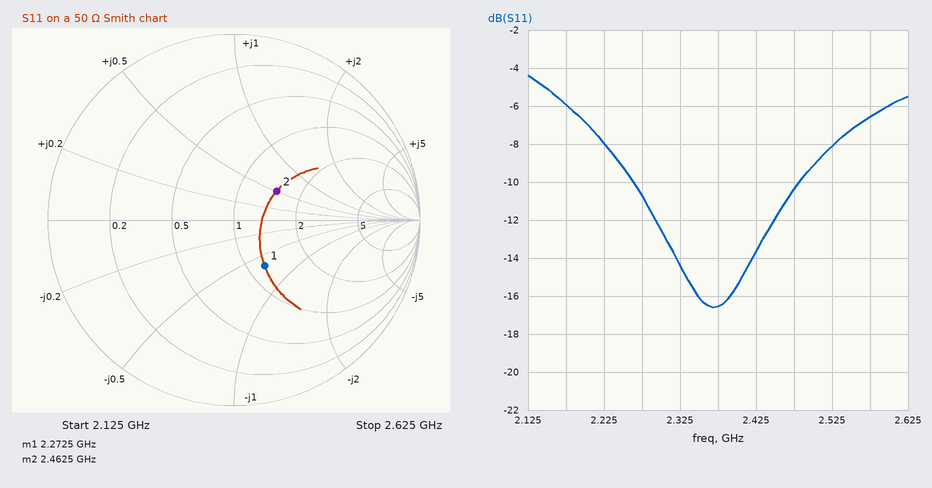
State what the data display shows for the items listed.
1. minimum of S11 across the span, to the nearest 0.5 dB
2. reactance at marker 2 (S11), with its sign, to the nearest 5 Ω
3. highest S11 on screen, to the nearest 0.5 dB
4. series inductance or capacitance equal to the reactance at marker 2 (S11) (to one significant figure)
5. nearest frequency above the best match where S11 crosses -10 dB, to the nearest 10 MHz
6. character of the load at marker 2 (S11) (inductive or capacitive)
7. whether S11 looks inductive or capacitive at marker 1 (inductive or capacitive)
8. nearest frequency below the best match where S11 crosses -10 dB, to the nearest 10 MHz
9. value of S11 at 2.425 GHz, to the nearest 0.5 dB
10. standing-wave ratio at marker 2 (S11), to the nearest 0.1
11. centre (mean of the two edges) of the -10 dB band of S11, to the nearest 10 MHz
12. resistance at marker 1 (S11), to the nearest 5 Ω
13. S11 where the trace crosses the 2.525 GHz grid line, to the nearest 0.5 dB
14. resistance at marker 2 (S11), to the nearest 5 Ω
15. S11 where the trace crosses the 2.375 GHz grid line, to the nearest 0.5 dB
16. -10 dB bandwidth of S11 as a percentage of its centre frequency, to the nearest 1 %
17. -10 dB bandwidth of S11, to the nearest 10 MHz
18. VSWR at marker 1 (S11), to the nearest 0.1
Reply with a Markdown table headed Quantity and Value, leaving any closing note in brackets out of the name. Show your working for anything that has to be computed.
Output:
| Quantity | Value |
|---|---|
| minimum of S11 across the span, to the nearest 0.5 dB | -16.5 dB |
| reactance at marker 2 (S11), with its sign, to the nearest 5 Ω | +25 Ω |
| highest S11 on screen, to the nearest 0.5 dB | -4.5 dB |
| series inductance or capacitance equal to the reactance at marker 2 (S11) | L = 25 Ω/(2π × 2.4625 GHz) ≈ 2 nH |
| nearest frequency above the best match where S11 crosses -10 dB, to the nearest 10 MHz | 2.48 GHz |
| character of the load at marker 2 (S11) | inductive |
| whether S11 looks inductive or capacitive at marker 1 | capacitive |
| nearest frequency below the best match where S11 crosses -10 dB, to the nearest 10 MHz | 2.26 GHz |
| value of S11 at 2.425 GHz, to the nearest 0.5 dB | -13.5 dB |
| standing-wave ratio at marker 2 (S11), to the nearest 0.1 | 1.8 |
| centre (mean of the two edges) of the -10 dB band of S11, to the nearest 10 MHz | 2.37 GHz |
| resistance at marker 1 (S11), to the nearest 5 Ω | 60 Ω |
| S11 where the trace crosses the 2.525 GHz grid line, to the nearest 0.5 dB | -8.0 dB |
| resistance at marker 2 (S11), to the nearest 5 Ω | 75 Ω |
| S11 where the trace crosses the 2.375 GHz grid line, to the nearest 0.5 dB | -16.5 dB |
| -10 dB bandwidth of S11 as a percentage of its centre frequency, to the nearest 1 % | 220 MHz / 2.37 GHz ≈ 9 % |
| -10 dB bandwidth of S11, to the nearest 10 MHz | 2.48 GHz − 2.26 GHz = 220 MHz |
| VSWR at marker 1 (S11), to the nearest 0.1 | 1.8 |
